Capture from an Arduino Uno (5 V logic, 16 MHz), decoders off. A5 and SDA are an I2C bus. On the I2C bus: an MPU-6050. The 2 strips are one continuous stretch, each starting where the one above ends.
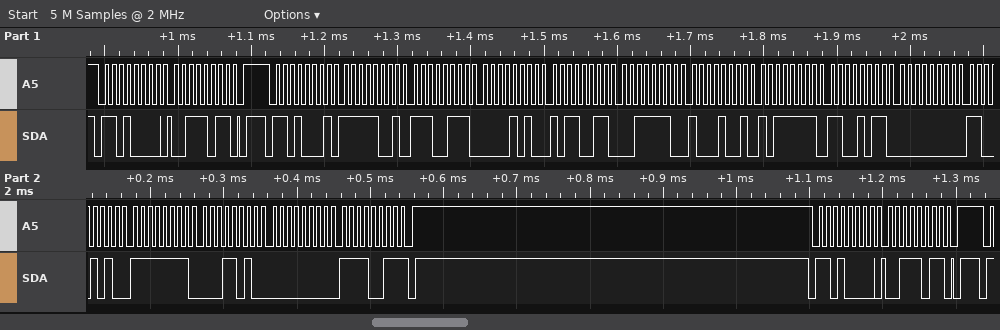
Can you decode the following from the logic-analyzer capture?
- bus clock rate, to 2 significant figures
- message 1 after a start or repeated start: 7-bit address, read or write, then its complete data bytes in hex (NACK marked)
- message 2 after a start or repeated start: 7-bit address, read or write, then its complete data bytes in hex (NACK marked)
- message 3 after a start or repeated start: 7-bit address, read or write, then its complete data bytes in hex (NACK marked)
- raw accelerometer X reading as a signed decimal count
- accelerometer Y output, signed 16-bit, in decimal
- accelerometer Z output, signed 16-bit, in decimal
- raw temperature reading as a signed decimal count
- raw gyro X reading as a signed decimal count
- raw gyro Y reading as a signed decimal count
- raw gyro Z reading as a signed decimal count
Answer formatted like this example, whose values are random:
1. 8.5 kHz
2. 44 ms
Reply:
1. 100 kHz
2. 0x68 write: 3B
3. 0x68 read: F9 E7 0A B3 3E 89 BF CB 00 CA FF 1A 00 F3 NACK
4. 0x68 write: 3B
5. -1561
6. 2739
7. 16009
8. -16437
9. 202
10. -230
11. 243
